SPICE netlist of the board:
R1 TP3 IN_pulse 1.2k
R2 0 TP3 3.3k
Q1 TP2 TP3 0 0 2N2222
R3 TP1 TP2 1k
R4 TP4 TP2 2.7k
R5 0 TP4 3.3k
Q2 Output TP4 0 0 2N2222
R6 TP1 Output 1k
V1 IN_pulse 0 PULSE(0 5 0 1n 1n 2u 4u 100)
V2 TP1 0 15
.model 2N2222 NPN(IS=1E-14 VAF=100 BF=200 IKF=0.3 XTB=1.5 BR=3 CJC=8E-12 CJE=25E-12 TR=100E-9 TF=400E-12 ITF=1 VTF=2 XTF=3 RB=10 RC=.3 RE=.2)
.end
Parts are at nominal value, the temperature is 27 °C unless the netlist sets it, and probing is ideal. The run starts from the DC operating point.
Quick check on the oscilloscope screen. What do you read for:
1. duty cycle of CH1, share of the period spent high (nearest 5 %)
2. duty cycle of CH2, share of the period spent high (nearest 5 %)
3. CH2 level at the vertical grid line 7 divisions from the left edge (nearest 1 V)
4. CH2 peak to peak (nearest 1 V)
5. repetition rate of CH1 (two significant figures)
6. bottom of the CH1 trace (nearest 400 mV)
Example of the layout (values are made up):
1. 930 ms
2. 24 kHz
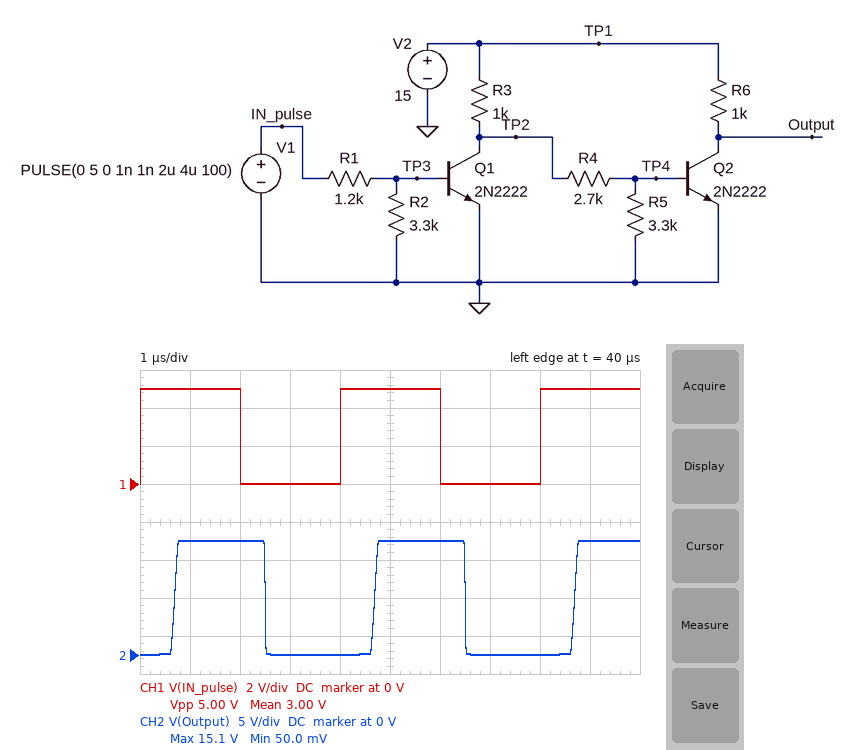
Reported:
1. 50 %
2. 45 %
3. 0 V
4. 15 V
5. 250 kHz
6. 0 V
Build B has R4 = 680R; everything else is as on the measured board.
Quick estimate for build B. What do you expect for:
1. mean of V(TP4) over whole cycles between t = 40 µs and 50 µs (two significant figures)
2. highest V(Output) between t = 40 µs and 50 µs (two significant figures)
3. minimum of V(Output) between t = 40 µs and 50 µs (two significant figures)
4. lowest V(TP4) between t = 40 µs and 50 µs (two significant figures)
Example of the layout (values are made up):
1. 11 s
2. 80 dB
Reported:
1. 460 mV
2. 15 V
3. 21 mV
4. 28 mV
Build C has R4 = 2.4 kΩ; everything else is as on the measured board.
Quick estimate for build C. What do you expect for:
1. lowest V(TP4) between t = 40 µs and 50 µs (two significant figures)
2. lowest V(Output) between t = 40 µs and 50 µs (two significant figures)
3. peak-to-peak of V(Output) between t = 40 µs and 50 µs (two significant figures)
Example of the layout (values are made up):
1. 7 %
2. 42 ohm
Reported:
1. 20 mV
2. 31 mV
3. 15 V
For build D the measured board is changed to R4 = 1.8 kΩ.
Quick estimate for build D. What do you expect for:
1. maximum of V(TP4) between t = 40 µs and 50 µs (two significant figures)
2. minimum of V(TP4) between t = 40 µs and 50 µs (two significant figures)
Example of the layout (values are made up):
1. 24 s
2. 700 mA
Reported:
1. 800 mV
2. 23 mV
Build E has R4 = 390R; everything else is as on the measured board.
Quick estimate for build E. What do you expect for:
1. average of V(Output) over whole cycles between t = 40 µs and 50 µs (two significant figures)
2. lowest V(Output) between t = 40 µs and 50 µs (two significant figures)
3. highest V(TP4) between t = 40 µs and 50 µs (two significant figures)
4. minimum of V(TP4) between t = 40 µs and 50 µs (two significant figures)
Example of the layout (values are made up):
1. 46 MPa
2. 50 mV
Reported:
1. 7.2 V
2. 18 mV
3. 870 mV
4. 30 mV
